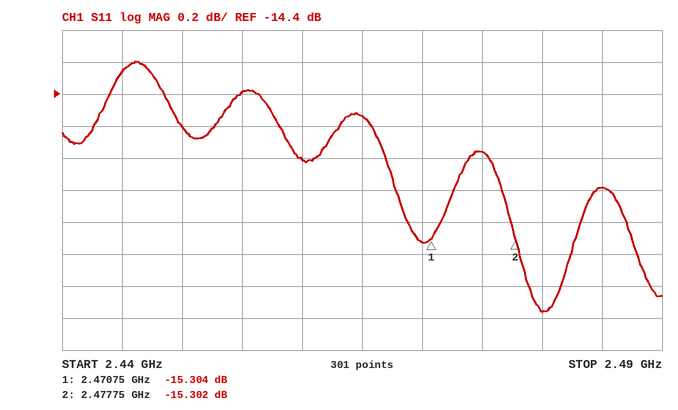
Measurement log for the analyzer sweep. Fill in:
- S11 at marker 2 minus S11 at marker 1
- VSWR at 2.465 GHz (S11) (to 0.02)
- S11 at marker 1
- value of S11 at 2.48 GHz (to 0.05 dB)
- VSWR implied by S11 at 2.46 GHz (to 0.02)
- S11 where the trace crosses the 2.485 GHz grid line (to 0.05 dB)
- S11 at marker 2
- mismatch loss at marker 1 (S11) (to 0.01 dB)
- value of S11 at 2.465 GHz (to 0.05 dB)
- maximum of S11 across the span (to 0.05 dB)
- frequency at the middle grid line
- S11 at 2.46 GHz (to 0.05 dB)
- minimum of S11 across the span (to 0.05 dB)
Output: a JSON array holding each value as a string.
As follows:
["0.002 dB", "1.46", "-15.304 dB", "-15.75 dB", "1.44", "-15.00 dB", "-15.302 dB", "0.13 dB", "-14.55 dB", "-14.20 dB", "2.465 GHz", "-14.80 dB", "-15.75 dB"]
